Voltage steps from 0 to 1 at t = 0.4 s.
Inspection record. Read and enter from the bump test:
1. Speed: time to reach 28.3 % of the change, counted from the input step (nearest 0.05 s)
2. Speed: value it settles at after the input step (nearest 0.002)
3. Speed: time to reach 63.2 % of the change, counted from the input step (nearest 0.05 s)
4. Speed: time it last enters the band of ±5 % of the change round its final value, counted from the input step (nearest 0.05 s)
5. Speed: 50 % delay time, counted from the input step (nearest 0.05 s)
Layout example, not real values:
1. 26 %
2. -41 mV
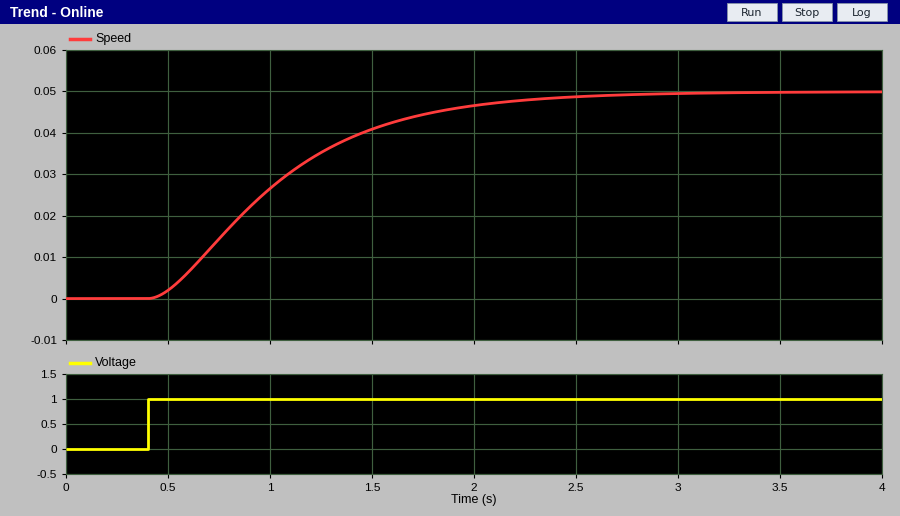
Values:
1. 0.35 s
2. 0.050
3. 0.75 s
4. 1.75 s
5. 0.55 s
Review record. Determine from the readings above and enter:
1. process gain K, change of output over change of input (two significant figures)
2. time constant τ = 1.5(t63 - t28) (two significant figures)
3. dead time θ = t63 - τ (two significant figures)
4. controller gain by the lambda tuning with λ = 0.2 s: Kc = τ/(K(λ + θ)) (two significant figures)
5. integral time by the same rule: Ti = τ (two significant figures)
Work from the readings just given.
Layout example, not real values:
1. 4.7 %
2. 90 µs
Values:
1. 0.050
2. 0.60 s
3. 0.15 s
4. 34
5. 0.60 s
